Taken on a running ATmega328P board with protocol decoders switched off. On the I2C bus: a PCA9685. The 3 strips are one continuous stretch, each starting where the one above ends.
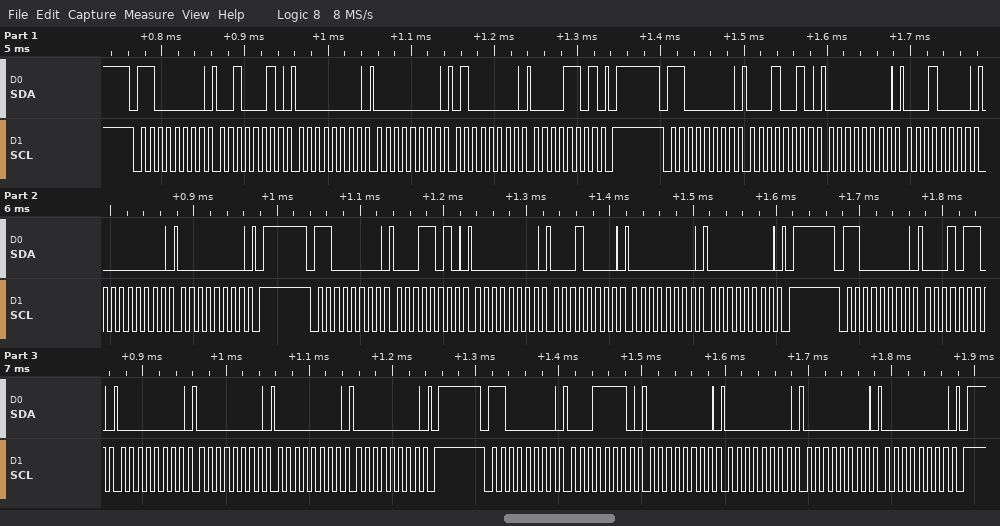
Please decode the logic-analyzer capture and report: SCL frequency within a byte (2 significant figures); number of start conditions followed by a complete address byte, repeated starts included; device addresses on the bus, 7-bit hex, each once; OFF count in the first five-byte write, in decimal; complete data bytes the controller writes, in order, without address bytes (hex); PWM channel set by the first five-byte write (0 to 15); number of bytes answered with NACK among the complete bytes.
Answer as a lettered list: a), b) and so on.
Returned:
a) 100 kHz
b) 5
c) 0x60
d) 3392
e) 22 00 00 40 0D 12 00 10 00 00 1A 00 10 00 00 16 00 00 00 00 1E 00 00 00 00
f) 7
g) 0
